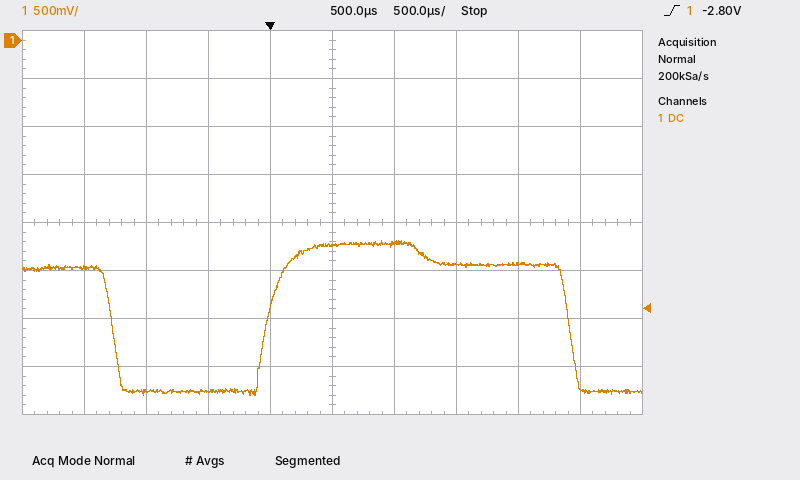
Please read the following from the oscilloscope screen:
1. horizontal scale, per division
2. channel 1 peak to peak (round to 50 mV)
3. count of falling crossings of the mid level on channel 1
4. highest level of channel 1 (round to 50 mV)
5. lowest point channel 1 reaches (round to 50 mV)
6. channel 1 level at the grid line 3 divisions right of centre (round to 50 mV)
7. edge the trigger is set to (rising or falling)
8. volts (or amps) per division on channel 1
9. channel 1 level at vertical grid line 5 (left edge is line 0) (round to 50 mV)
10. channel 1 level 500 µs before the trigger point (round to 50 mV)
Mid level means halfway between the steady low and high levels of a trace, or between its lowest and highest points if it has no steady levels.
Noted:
500 µs
1.60 V
2
-2.10 V
-3.70 V
-2.35 V
rising
500 mV
-2.15 V
-3.65 V
